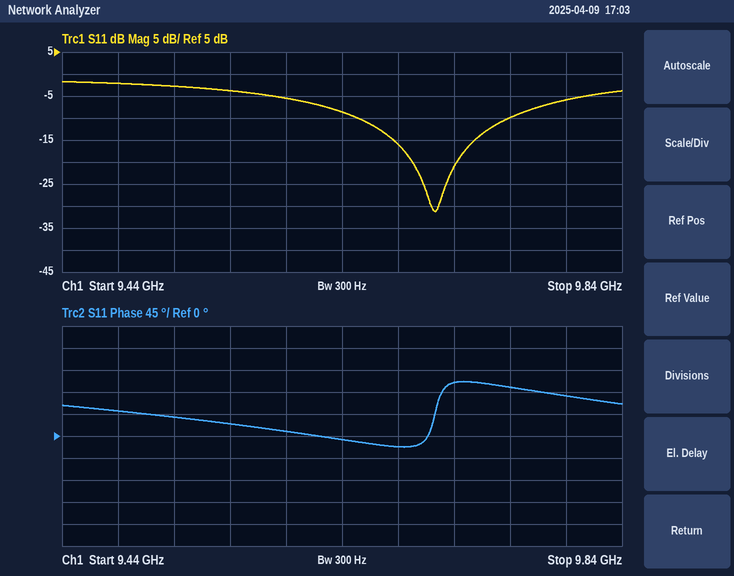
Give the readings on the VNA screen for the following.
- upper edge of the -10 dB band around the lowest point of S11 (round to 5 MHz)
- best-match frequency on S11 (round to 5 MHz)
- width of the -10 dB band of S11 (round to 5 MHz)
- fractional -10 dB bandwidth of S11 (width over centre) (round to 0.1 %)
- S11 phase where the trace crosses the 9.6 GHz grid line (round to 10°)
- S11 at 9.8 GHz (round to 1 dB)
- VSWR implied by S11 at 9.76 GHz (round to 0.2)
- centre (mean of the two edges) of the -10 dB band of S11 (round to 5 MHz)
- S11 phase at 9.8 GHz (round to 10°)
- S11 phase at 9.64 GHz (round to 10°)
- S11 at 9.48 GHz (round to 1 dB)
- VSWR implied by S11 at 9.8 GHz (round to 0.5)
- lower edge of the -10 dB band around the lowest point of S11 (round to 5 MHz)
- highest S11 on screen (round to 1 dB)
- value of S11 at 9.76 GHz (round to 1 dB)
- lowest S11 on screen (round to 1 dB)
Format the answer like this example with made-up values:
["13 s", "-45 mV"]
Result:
["9.760 GHz", "9.705 GHz", "110 MHz", "1.1 %", "10°", "-6 dB", "2.0", "9.705 GHz", "80°", "-10°", "-2 dB", "3.0", "9.650 GHz", "-2 dB", "-10 dB", "-31 dB"]
